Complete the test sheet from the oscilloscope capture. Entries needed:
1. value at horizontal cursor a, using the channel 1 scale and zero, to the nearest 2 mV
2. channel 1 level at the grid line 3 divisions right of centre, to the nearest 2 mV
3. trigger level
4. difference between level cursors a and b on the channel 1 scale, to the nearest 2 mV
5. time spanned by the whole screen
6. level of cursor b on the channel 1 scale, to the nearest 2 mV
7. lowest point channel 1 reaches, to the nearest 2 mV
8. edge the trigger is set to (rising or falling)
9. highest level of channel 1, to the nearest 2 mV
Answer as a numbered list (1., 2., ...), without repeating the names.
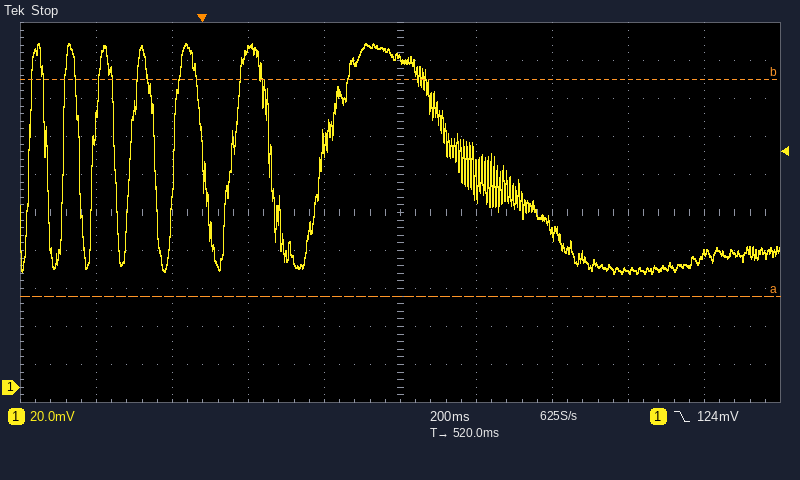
1. 48 mV
2. 62 mV
3. 124 mV
4. 114 mV
5. 2 s
6. 162 mV
7. 60 mV
8. falling
9. 180 mV
